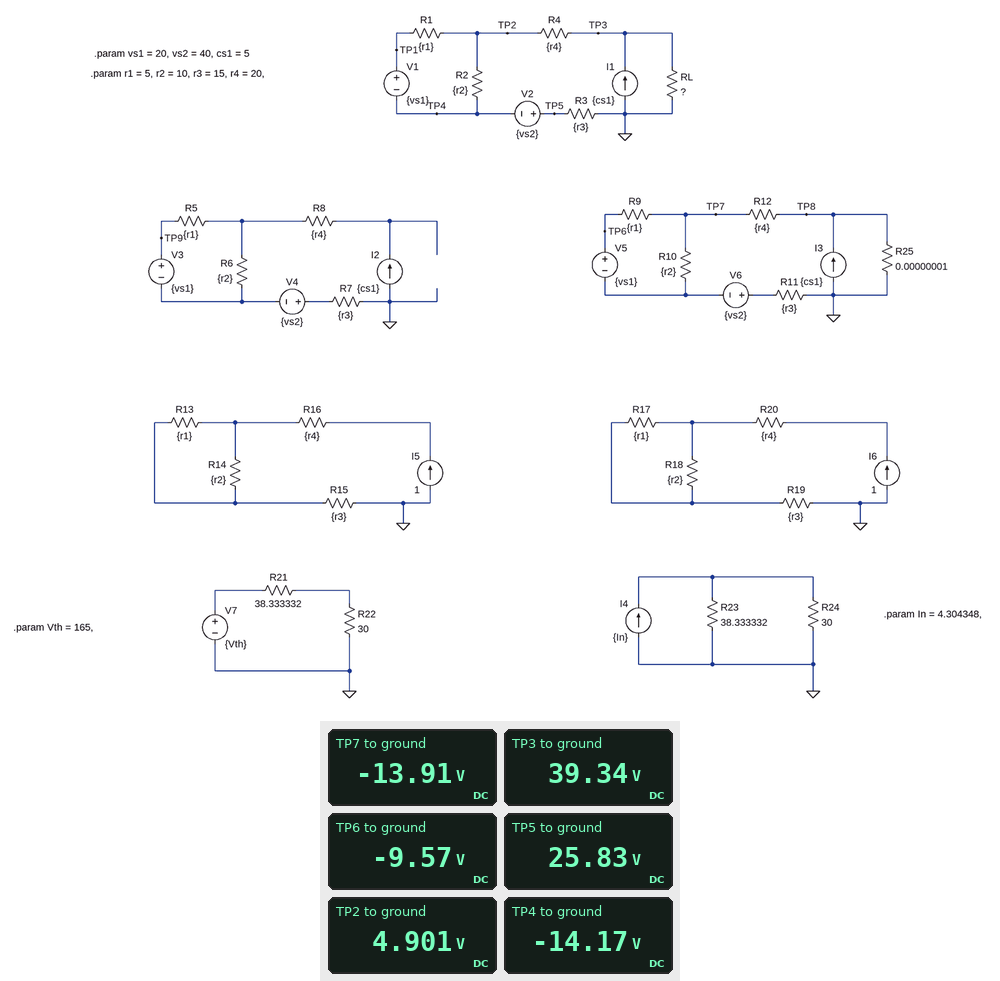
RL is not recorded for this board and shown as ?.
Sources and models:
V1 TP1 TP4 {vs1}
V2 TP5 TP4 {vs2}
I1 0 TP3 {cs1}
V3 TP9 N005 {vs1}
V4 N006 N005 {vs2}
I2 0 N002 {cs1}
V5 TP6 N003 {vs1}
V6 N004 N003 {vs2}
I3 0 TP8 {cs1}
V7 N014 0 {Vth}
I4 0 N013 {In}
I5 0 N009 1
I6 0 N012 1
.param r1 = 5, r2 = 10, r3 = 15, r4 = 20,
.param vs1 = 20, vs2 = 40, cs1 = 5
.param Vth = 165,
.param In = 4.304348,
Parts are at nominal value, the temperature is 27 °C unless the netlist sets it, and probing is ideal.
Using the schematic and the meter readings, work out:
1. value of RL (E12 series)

12 Ω
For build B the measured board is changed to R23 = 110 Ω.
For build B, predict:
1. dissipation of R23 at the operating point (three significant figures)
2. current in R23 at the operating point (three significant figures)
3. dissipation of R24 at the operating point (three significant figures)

93.6 W
922 mA
343 W
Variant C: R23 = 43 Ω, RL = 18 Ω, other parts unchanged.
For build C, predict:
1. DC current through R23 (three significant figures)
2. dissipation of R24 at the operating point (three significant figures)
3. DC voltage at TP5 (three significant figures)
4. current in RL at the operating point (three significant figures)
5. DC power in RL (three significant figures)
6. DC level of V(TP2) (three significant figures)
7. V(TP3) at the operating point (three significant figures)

1.77 A
193 W
31.1 V
2.93 A
154 W
11.3 V
52.7 V
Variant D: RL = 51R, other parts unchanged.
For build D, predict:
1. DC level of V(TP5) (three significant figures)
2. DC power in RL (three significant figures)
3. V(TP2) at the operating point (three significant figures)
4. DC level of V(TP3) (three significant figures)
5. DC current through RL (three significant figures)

47.3 V
174 W
31.1 V
94.2 V
1.85 A
